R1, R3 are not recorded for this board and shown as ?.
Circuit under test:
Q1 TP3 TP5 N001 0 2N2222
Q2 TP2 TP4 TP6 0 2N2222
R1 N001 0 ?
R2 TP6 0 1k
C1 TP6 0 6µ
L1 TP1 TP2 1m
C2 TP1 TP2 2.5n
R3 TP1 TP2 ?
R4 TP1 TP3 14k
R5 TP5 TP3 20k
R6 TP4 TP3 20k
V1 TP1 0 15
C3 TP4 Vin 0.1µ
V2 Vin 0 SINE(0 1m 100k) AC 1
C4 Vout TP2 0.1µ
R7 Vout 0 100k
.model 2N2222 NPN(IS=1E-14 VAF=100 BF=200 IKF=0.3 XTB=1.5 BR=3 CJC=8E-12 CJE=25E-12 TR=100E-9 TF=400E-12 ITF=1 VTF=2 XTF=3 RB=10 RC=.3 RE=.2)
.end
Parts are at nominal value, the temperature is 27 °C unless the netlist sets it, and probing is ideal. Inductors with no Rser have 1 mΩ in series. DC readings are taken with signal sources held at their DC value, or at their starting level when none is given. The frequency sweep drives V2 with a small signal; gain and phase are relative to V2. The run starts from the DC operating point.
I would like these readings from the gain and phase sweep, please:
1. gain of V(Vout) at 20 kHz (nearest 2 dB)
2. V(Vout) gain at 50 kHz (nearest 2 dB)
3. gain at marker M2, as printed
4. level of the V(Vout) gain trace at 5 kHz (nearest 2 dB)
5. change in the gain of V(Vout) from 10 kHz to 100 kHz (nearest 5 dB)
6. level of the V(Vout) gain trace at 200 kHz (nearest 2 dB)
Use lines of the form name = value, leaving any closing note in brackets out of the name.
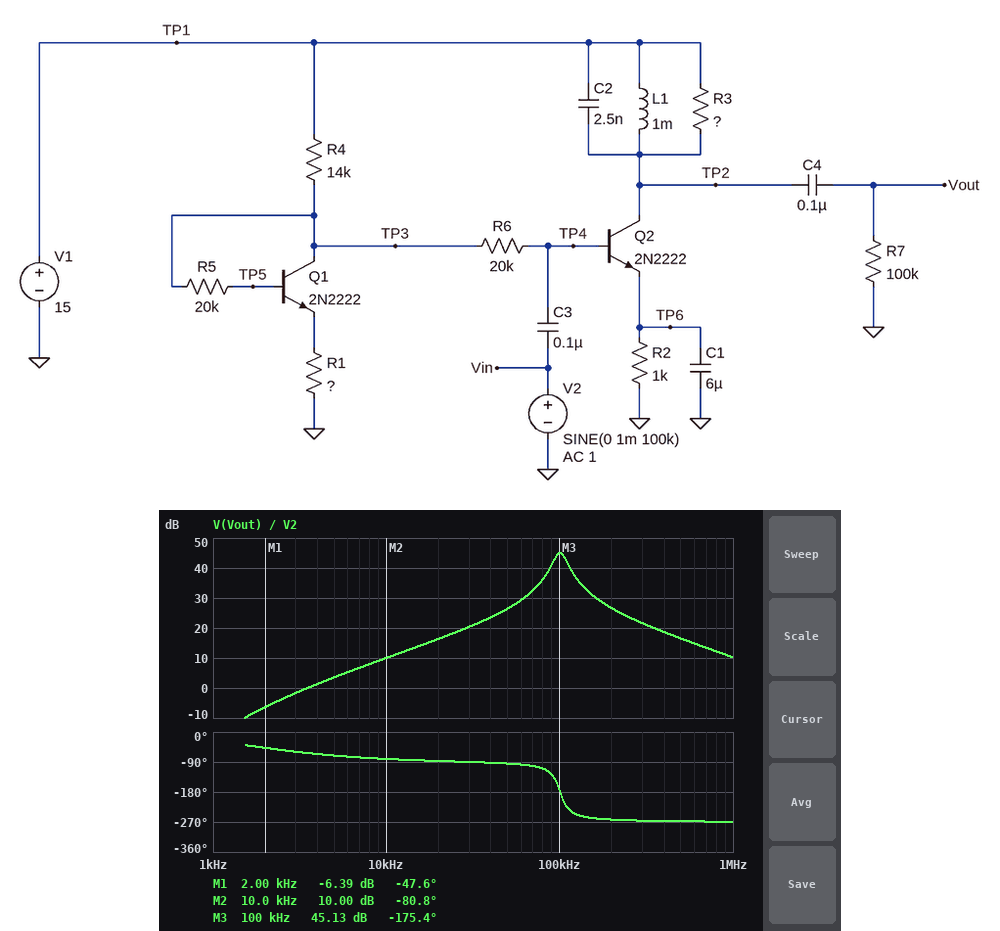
gain of V(Vout) at 20 kHz = 16 dB
V(Vout) gain at 50 kHz = 26 dB
gain at marker M2, as printed = 10.00 dB
level of the V(Vout) gain trace at 5 kHz = 4 dB
change in the gain of V(Vout) from 10 kHz to 100 kHz = 35 dB
level of the V(Vout) gain trace at 200 kHz = 26 dB
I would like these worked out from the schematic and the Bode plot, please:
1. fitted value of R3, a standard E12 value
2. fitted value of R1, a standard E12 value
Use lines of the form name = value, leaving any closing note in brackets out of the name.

fitted value of R3, a standard E12 value = 3.9 kΩ
fitted value of R1, a standard E12 value = 1.5 kΩ
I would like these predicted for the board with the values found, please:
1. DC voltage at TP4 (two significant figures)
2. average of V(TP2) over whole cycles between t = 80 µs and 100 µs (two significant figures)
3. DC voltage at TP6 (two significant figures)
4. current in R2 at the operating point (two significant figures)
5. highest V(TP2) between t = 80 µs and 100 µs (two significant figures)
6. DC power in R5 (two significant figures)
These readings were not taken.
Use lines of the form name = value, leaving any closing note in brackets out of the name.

DC voltage at TP4 = 2.0 V
average of V(TP2) over whole cycles between t = 80 µs and 100 µs = 15 V
DC voltage at TP6 = 1.3 V
current in R2 at the operating point = 1.3 mA
highest V(TP2) between t = 80 µs and 100 µs = 15 V
DC power in R5 = 420 nW
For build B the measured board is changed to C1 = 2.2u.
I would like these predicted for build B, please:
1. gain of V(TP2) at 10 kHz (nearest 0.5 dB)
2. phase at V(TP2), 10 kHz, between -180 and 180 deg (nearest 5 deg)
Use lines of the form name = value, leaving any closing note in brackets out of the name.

gain of V(TP2) at 10 kHz = 9.5 dB
phase at V(TP2), 10 kHz, between -180 and 180 deg = -70 deg
